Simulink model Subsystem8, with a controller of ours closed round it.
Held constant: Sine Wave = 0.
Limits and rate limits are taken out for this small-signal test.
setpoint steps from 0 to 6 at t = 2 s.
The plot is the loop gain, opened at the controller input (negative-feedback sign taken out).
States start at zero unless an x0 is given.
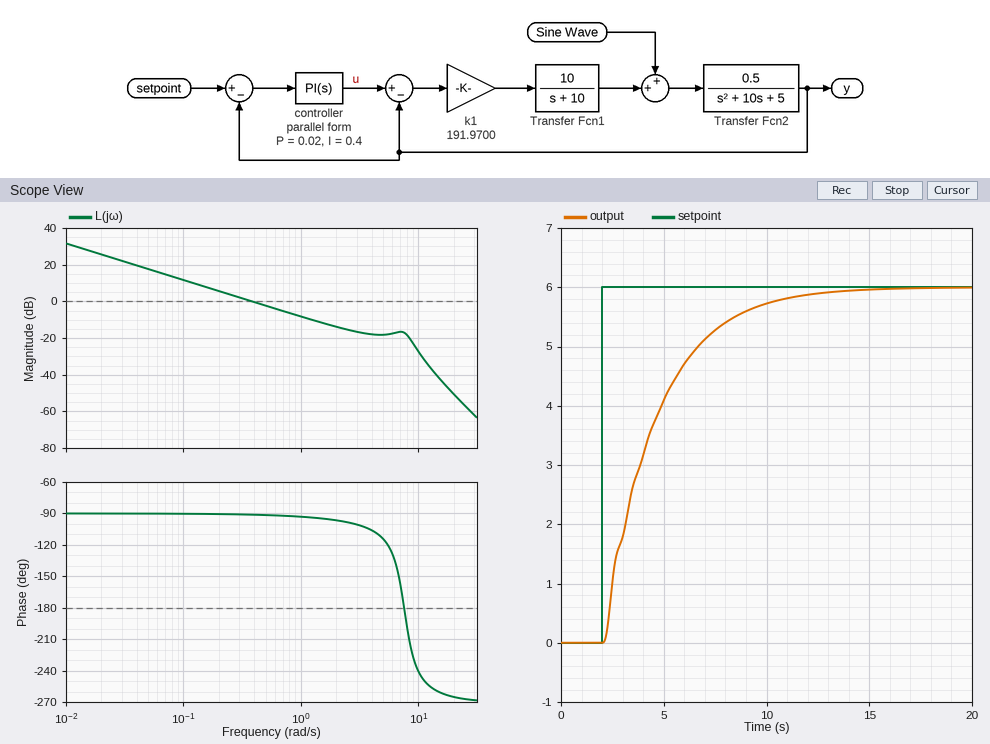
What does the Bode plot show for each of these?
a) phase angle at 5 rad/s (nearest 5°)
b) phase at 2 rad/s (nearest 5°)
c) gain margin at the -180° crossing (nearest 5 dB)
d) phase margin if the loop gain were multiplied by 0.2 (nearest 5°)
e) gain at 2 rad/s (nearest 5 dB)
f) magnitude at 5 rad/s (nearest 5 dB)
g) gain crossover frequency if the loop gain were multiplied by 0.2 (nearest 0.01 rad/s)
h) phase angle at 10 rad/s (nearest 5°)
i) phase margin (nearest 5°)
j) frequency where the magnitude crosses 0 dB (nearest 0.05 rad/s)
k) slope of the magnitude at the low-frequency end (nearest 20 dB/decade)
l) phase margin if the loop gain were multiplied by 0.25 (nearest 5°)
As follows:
-115°
-95°
15 dB
90°
-15 dB
-20 dB
0.08 rad/s
-240°
90°
0.40 rad/s
-20 dB/decade
90°
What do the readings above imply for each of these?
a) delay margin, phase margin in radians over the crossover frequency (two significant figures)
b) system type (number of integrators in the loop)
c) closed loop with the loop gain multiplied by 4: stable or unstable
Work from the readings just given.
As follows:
3.9 s
1
stable
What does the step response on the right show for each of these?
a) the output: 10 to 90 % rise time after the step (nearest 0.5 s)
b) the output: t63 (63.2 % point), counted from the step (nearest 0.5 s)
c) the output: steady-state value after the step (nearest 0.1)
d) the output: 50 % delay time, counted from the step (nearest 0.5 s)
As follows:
5.5 s
2.5 s
6.0
2.0 s
